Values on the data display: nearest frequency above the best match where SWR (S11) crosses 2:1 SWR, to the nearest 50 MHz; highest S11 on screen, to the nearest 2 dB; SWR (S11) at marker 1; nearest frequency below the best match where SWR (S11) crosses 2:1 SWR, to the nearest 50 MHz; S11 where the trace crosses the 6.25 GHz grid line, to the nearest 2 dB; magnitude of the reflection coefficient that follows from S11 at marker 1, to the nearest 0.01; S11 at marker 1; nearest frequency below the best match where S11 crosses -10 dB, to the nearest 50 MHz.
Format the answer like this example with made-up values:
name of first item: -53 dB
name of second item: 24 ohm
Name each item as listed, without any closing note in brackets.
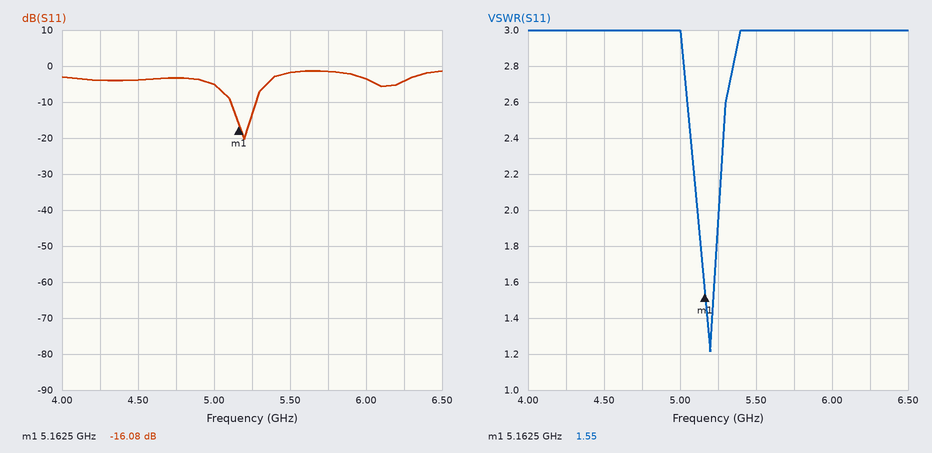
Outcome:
nearest frequency above the best match where SWR (S11) crosses 2:1 SWR, to the nearest 50 MHz: 5.25 GHz
highest S11 on screen, to the nearest 2 dB: -2 dB
SWR (S11) at marker 1: 1.55
nearest frequency below the best match where SWR (S11) crosses 2:1 SWR, to the nearest 50 MHz: 5.10 GHz
S11 where the trace crosses the 6.25 GHz grid line, to the nearest 2 dB: -4 dB
magnitude of the reflection coefficient that follows from S11 at marker 1, to the nearest 0.01: 0.16
S11 at marker 1: -16.08 dB
nearest frequency below the best match where S11 crosses -10 dB, to the nearest 50 MHz: 5.10 GHz
